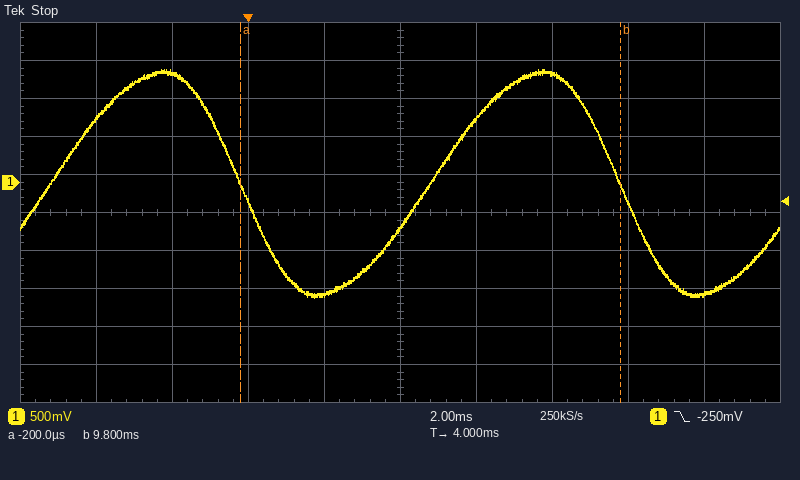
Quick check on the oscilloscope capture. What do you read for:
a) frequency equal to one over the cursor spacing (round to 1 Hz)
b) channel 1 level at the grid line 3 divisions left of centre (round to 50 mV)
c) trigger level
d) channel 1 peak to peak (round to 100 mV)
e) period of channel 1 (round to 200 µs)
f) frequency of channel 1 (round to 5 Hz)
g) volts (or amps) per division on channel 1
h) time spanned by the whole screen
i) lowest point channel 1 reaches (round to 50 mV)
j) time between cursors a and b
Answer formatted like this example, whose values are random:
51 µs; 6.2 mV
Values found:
100 Hz; 1.45 V; -250 mV; 3.00 V; 10.0 ms; 100 Hz; 500 mV; 20 ms; -1.50 V; 10.0 ms
